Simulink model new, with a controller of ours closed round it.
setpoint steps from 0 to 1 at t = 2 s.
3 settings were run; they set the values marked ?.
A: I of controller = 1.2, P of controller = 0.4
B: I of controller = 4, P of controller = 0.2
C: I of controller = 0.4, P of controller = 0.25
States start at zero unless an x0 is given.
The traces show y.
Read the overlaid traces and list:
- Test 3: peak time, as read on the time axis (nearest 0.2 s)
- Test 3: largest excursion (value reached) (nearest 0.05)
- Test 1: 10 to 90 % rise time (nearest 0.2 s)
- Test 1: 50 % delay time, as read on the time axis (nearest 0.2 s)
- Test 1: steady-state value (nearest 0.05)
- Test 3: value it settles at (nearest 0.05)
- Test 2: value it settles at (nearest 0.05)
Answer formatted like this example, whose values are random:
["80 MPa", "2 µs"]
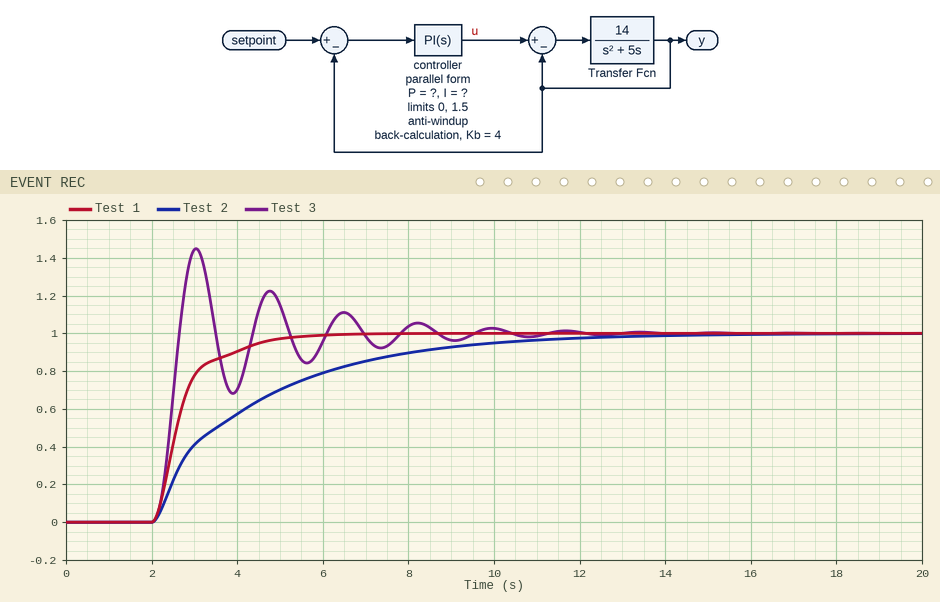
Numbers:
["3.0 s", "1.45", "1.8 s", "2.6 s", "1.00", "1.00", "1.00"]
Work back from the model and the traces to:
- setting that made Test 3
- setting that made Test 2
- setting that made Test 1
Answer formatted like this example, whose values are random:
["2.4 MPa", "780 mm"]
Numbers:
["B", "C", "A"]
